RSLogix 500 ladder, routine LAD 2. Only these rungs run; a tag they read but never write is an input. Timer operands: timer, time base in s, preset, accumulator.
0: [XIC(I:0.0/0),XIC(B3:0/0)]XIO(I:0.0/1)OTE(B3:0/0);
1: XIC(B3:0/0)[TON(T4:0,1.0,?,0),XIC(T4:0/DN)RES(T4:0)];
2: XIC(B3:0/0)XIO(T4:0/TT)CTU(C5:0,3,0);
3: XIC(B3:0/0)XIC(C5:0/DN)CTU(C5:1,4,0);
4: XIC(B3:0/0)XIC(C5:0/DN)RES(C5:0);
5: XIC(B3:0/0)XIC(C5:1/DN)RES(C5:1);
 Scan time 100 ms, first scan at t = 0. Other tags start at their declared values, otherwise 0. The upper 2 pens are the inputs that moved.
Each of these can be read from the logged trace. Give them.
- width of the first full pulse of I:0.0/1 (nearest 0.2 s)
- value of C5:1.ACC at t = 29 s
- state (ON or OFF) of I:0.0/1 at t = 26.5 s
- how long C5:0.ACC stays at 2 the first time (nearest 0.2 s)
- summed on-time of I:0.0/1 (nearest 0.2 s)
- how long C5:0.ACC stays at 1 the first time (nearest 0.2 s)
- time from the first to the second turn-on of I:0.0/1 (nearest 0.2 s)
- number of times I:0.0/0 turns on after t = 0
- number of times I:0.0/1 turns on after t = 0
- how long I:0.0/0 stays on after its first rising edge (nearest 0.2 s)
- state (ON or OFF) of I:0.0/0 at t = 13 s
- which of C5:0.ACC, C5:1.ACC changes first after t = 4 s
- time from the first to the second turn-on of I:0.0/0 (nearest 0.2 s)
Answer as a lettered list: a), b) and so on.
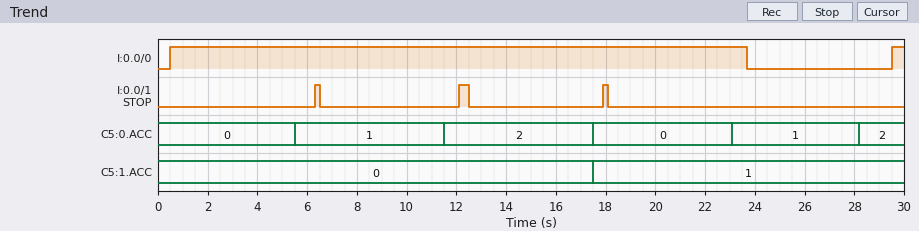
a) 0.2 s
b) 1
c) OFF
d) 6.0 s
e) 0.8 s
f) 6.0 s
g) 5.8 s
h) 2
i) 3
j) 23.2 s
k) ON
l) C5:0.ACC
m) 29.0 s
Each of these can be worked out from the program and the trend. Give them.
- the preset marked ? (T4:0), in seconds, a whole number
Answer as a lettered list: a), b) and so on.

a) 5 s
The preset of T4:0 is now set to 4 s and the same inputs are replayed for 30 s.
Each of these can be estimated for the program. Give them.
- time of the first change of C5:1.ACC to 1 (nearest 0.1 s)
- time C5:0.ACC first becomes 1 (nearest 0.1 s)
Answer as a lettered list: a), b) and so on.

a) 16.5 s
b) 4.5 s
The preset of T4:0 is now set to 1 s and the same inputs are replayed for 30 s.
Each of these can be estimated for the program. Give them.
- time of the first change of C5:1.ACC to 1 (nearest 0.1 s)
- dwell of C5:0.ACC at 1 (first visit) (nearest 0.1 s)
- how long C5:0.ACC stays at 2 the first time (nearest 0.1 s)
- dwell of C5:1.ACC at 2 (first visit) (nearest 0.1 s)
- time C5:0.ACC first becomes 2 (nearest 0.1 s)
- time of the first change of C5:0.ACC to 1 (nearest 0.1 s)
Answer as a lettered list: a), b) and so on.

a) 3.7 s
b) 1.1 s
c) 1.1 s
d) 3.3 s
e) 2.6 s
f) 1.5 s
